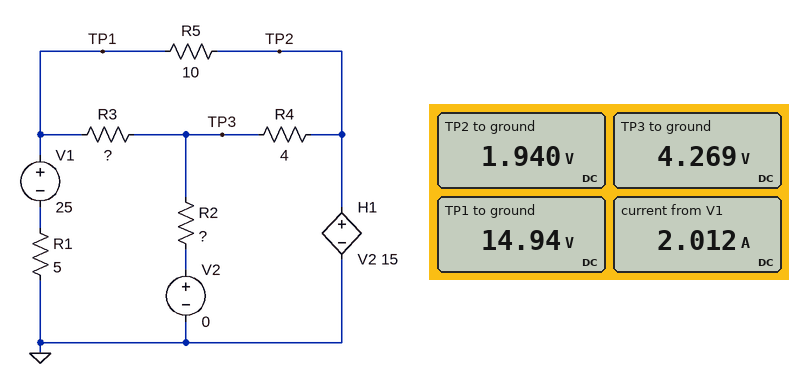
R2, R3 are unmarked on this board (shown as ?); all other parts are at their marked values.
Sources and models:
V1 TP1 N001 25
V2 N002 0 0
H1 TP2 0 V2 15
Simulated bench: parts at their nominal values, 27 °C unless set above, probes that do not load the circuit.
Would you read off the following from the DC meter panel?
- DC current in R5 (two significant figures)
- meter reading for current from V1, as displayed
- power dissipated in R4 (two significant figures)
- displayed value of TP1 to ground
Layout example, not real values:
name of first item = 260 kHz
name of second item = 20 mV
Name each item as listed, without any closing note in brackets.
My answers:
DC current in R5 = 1.3 A
meter reading for current from V1, as displayed = 2.012 A
power dissipated in R4 = 1.4 W
displayed value of TP1 to ground = 14.94 V
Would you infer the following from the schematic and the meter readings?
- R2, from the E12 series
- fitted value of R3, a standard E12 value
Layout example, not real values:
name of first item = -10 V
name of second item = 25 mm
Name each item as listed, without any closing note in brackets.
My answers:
R2, from the E12 series = 33 Ω
fitted value of R3, a standard E12 value = 15 Ω
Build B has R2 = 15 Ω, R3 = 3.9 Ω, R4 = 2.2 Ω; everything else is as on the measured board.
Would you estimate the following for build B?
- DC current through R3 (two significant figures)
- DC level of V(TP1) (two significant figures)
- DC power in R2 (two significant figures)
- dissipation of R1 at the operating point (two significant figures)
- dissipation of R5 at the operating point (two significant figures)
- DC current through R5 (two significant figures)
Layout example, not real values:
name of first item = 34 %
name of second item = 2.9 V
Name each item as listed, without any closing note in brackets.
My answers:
DC current through R3 = 970 mA
DC level of V(TP1) = 18 V
DC power in R2 = 14 W
dissipation of R1 at the operating point = 9.0 W
dissipation of R5 at the operating point = 1.4 W
DC current through R5 = 380 mA
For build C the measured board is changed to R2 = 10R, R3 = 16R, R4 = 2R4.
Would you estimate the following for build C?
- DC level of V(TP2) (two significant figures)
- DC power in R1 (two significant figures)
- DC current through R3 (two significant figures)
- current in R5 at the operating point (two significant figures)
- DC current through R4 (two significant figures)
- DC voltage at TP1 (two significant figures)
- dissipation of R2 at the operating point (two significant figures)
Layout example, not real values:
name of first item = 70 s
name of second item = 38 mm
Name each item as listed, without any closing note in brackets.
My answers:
DC level of V(TP2) = -16 V
DC power in R1 = 60 W
DC current through R3 = 1.1 A
current in R5 at the operating point = 2.3 A
DC current through R4 = 2.2 A
DC voltage at TP1 = 7.7 V
dissipation of R2 at the operating point = 11 W
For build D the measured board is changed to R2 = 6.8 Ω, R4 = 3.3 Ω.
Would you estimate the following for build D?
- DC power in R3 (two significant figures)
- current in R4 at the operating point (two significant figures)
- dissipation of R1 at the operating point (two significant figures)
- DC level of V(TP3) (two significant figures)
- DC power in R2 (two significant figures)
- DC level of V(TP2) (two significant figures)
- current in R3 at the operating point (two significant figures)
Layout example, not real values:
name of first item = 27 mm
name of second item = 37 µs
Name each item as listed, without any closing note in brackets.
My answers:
DC power in R3 = 14 W
current in R4 at the operating point = 1.6 A
dissipation of R1 at the operating point = 44 W
DC level of V(TP3) = -4.5 V
DC power in R2 = 2.9 W
DC level of V(TP2) = -9.8 V
current in R3 at the operating point = 970 mA
